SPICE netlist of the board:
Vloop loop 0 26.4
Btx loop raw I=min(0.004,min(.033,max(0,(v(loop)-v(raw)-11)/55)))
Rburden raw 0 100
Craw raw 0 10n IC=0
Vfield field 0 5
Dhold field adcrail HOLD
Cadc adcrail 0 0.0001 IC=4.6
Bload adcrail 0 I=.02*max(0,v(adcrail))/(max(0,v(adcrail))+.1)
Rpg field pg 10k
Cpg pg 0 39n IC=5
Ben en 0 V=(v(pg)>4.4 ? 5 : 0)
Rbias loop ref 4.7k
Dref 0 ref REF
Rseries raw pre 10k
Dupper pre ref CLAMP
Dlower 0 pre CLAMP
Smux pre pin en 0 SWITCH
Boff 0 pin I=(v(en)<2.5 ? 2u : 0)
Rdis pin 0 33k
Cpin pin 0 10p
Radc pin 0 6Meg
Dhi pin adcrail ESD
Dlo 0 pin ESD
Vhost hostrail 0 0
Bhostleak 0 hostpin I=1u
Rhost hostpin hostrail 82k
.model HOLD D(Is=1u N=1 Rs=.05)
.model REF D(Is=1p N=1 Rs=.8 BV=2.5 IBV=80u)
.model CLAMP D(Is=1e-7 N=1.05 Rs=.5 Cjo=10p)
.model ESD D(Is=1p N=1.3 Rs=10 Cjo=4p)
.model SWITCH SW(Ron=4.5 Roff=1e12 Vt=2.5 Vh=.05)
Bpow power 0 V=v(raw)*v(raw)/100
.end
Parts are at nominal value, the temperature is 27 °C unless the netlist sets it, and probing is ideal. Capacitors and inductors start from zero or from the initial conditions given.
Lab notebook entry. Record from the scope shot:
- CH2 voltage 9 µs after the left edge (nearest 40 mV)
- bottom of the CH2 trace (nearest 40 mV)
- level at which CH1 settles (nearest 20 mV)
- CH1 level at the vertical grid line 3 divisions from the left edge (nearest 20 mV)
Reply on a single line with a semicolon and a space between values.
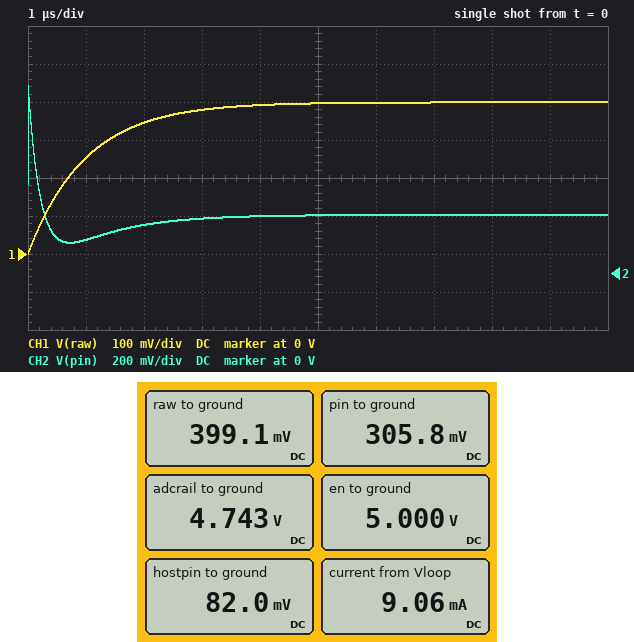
320 mV; 160 mV; 400 mV; 380 mV
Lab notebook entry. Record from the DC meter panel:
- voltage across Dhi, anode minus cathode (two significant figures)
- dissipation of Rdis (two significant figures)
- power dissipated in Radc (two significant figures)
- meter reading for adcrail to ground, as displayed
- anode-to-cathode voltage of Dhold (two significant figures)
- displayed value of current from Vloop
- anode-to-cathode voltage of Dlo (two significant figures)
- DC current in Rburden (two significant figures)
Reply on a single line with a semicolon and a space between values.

-4.4 V; 2.8 µW; 16 nW; 4.743 V; 260 mV; 9.06 mA; -310 mV; 4.0 mA
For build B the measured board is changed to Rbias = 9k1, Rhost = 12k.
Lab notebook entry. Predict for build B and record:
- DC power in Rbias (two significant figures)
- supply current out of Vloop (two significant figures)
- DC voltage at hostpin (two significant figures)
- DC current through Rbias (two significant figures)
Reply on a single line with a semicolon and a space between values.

62 mW; 6.6 mA; 12 mV; 2.6 mA
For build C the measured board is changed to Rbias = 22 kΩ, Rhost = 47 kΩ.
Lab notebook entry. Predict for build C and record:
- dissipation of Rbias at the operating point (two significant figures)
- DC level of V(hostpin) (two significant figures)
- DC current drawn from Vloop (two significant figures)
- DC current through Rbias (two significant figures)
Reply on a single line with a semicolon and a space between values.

26 mW; 47 mV; 5.1 mA; 1.1 mA
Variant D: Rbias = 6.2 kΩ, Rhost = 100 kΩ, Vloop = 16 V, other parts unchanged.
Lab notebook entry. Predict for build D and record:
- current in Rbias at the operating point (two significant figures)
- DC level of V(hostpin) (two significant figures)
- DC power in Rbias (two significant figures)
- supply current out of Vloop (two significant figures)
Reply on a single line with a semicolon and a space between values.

2.2 mA; 100 mV; 29 mW; 6.2 mA
